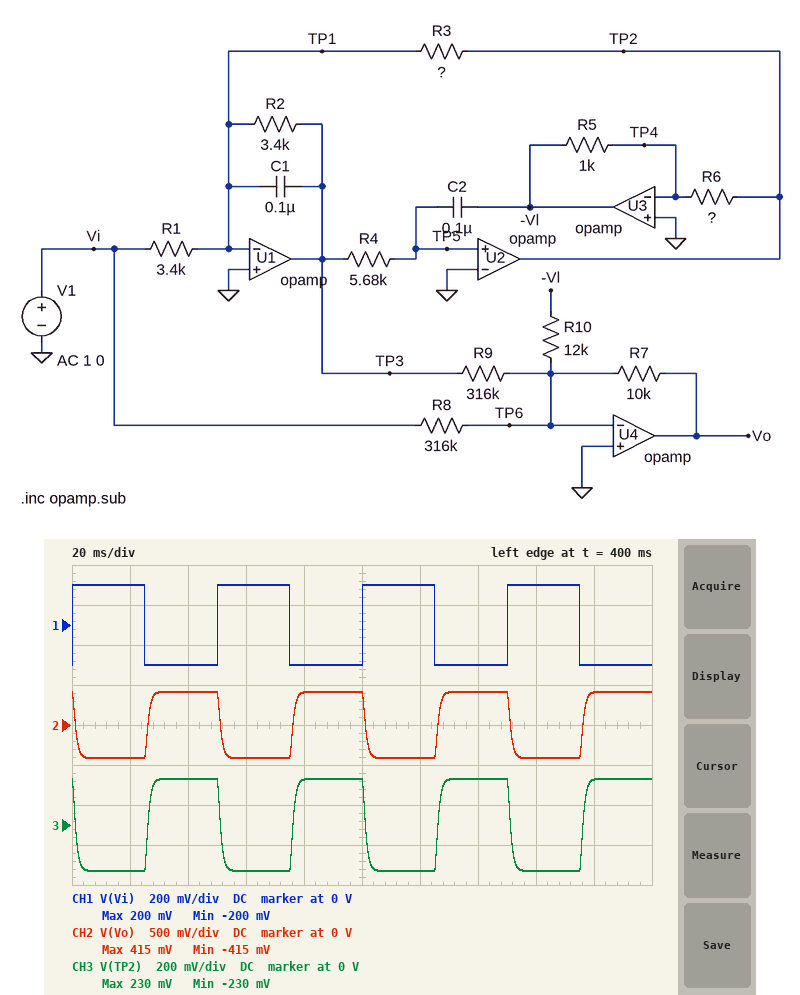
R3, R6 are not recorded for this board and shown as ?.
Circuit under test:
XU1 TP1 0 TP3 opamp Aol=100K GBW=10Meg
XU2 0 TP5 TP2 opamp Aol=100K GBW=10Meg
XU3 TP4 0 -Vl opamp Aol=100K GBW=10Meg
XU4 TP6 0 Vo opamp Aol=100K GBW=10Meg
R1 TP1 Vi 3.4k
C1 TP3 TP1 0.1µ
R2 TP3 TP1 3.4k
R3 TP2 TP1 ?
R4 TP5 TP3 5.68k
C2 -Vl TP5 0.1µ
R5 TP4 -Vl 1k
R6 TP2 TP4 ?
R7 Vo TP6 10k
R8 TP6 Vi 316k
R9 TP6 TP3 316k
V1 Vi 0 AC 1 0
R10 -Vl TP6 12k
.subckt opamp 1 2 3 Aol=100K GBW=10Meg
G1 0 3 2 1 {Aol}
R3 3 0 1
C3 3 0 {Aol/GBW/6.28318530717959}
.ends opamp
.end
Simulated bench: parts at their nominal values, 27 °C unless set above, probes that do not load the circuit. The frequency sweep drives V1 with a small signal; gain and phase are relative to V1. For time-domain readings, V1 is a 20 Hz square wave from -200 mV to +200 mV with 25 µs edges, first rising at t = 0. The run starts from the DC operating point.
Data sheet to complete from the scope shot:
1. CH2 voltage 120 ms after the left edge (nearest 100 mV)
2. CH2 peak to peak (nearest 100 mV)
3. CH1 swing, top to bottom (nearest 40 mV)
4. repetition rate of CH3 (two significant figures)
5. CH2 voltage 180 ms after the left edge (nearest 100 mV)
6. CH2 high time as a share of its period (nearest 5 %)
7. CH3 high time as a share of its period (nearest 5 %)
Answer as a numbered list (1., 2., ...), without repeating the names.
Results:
1. -400 mV
2. 800 mV
3. 400 mV
4. 20 Hz
5. 400 mV
6. 50 %
7. 50 %
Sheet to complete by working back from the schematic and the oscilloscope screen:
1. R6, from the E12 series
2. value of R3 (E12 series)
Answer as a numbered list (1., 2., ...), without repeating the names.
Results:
1. 470 Ω
2. 3.9 kΩ
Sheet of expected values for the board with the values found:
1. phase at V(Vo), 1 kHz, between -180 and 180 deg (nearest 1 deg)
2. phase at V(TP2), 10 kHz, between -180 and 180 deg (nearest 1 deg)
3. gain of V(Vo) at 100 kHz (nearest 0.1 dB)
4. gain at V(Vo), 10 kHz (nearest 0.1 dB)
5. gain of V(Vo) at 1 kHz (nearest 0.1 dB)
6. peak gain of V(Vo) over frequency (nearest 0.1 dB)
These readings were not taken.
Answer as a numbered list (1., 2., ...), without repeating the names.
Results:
1. 26 deg
2. 3 deg
3. -30.0 dB
4. -30.3 dB
5. -22.5 dB
6. 6.3 dB
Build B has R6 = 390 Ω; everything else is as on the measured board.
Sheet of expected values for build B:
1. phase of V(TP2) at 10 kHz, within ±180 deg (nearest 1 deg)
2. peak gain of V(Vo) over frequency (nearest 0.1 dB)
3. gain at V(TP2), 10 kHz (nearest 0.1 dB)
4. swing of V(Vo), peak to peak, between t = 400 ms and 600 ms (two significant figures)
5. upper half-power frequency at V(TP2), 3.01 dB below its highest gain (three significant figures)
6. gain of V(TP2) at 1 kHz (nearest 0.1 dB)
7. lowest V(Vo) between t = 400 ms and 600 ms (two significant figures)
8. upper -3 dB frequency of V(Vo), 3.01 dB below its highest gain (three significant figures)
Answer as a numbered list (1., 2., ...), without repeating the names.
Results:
1. 3 deg
2. 7.9 dB
3. -65.8 dB
4. 990 mV
5. 118 Hz
6. -26.4 dB
7. -500 mV
8. 117 Hz
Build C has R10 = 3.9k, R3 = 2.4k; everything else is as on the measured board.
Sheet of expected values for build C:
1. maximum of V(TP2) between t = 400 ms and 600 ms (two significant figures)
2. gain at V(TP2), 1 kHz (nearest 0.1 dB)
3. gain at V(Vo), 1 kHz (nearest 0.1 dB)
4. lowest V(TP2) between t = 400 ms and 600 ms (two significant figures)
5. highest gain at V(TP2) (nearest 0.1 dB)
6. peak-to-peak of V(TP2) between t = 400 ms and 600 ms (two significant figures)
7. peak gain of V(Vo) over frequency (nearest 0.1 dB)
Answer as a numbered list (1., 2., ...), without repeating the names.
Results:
1. 150 mV
2. -24.4 dB
3. -10.5 dB
4. -150 mV
5. -3.0 dB
6. 290 mV
7. 11.8 dB
